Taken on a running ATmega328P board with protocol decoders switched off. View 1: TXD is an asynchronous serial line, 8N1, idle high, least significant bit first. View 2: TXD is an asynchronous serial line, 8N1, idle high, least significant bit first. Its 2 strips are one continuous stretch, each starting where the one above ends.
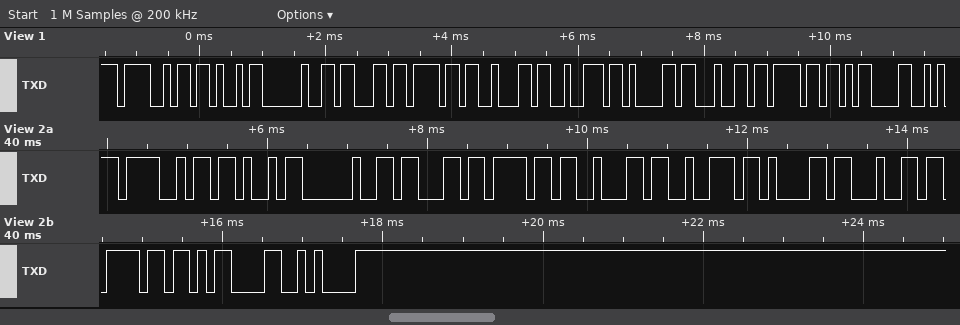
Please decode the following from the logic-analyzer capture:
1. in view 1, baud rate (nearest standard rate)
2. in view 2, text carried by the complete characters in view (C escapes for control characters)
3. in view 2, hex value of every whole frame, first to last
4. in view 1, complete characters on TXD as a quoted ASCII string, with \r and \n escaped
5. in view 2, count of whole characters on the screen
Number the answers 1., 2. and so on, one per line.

1. 9600 baud
2. "OK cobrado\r\n"
3. 4F 4B 20 63 6F 62 72 61 64 6F 0D 0A
4. "OK cobrado\r"
5. 12
